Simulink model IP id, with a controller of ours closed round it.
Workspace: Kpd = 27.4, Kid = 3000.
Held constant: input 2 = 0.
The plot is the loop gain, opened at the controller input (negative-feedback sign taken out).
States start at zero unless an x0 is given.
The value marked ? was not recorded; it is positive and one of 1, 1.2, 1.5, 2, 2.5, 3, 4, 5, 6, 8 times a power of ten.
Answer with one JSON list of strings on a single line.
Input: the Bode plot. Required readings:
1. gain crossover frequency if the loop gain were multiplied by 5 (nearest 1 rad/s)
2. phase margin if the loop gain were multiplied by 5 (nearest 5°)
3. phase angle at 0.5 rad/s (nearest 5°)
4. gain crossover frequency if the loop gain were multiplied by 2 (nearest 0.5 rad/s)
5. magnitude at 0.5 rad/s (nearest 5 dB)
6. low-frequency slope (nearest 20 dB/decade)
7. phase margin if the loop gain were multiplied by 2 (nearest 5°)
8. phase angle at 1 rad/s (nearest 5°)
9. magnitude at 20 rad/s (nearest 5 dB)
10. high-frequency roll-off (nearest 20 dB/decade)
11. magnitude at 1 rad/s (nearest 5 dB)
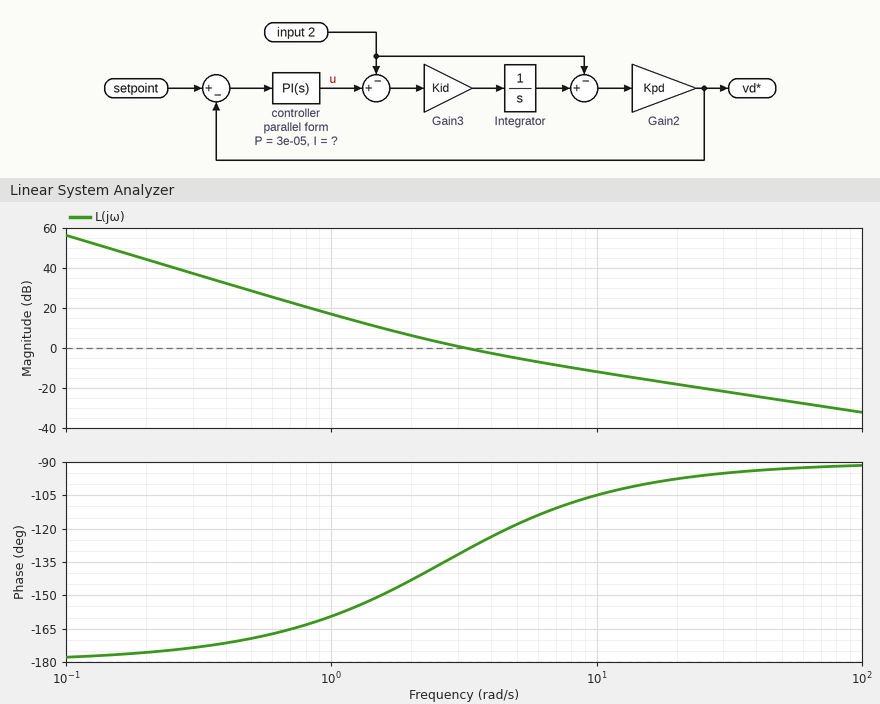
["13 rad/s", "80°", "-170°", "5.5 rad/s", "30 dB", "-40 dB/decade", "65°", "-160°", "-20 dB", "-20 dB/decade", "15 dB"]
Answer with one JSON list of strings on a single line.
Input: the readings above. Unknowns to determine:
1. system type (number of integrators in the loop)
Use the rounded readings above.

["2"]
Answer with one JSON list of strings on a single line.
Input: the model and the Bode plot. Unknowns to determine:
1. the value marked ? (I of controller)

["8e-05"]
